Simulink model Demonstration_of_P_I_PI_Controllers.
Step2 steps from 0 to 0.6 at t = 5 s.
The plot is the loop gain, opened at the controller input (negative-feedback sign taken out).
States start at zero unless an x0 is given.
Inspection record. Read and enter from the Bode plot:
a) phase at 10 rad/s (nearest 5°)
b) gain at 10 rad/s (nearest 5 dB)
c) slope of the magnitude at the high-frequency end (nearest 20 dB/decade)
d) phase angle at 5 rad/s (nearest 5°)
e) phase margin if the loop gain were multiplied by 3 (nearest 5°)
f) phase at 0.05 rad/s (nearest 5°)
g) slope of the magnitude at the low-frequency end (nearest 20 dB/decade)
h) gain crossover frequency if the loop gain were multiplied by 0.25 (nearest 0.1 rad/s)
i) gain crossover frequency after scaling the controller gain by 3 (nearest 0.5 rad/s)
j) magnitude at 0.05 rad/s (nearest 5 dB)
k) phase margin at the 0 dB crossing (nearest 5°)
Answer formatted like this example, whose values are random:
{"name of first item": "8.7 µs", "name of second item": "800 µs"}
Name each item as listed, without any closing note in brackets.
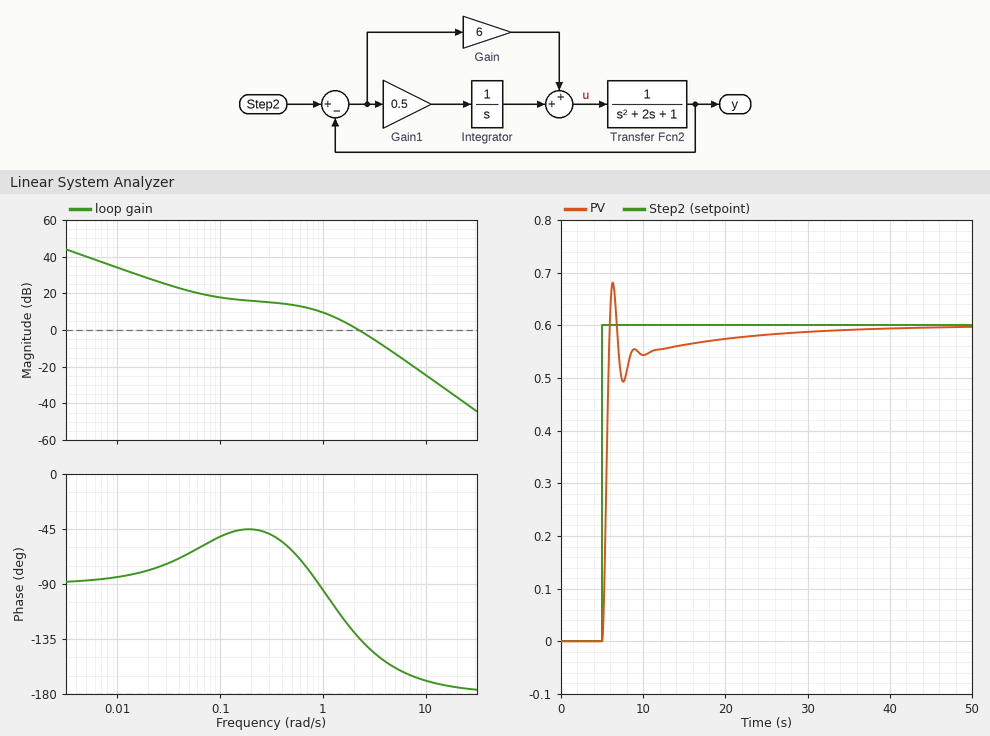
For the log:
{"phase at 10 rad/s": "-170°", "gain at 10 rad/s": "-25 dB", "slope of the magnitude at the high-frequency end": "-40 dB/decade", "phase angle at 5 rad/s": "-160°", "phase margin if the loop gain were multiplied by 3": "25°", "phase at 0.05 rad/s": "-65°", "slope of the magnitude at the low-frequency end": "-20 dB/decade", "gain crossover frequency if the loop gain were multiplied by 0.25": "0.7 rad/s", "gain crossover frequency after scaling the controller gain by 3": "4.0 rad/s", "magnitude at 0.05 rad/s": "20 dB", "phase margin at the 0 dB crossing": "45°"}
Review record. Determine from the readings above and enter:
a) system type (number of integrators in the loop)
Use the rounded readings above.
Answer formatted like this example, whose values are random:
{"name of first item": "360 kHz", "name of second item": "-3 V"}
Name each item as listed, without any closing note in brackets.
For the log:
{"system type": "1"}
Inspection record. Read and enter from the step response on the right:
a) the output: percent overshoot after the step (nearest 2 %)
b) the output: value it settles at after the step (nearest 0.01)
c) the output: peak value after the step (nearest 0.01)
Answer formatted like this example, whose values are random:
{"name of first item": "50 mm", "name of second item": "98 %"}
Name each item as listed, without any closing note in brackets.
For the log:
{"the output: percent overshoot after the step": "14 %", "the output: value it settles at after the step": "0.60", "the output: peak value after the step": "0.68"}
